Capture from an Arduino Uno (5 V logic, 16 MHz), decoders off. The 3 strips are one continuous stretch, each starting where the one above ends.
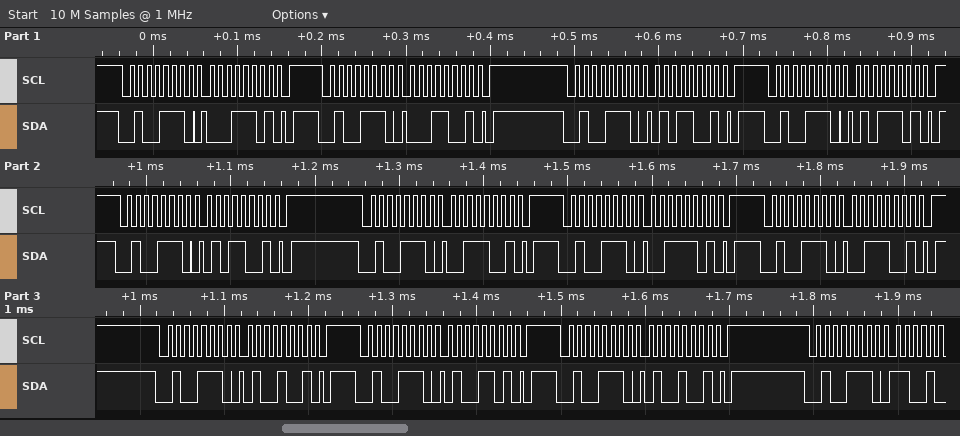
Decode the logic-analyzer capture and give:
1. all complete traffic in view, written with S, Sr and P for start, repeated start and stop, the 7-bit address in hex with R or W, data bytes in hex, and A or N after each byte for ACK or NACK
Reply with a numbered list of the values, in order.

1. S 27W A 1D A P S 27W A 19 A P S 27W A 59 A P S 27W A 5D A P S 27W A 59 A P S 27W A 39 A P S 27W A 3D A P S 27W A 39 A P S 27W A 49 A P S 27W A 4D A P S 27W A 49 A P S 27W A
